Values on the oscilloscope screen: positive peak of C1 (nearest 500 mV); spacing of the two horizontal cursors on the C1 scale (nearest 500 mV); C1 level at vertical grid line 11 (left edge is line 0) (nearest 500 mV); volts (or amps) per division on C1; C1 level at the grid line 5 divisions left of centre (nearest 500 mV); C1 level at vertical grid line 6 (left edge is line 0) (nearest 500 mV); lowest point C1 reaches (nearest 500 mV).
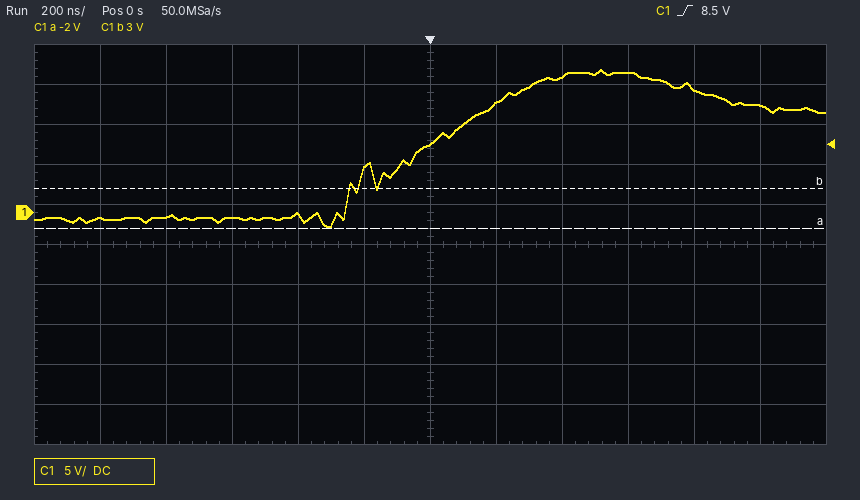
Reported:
18.0 V
5.0 V
13.5 V
5 V
-500 mV
8.5 V
-2.0 V
